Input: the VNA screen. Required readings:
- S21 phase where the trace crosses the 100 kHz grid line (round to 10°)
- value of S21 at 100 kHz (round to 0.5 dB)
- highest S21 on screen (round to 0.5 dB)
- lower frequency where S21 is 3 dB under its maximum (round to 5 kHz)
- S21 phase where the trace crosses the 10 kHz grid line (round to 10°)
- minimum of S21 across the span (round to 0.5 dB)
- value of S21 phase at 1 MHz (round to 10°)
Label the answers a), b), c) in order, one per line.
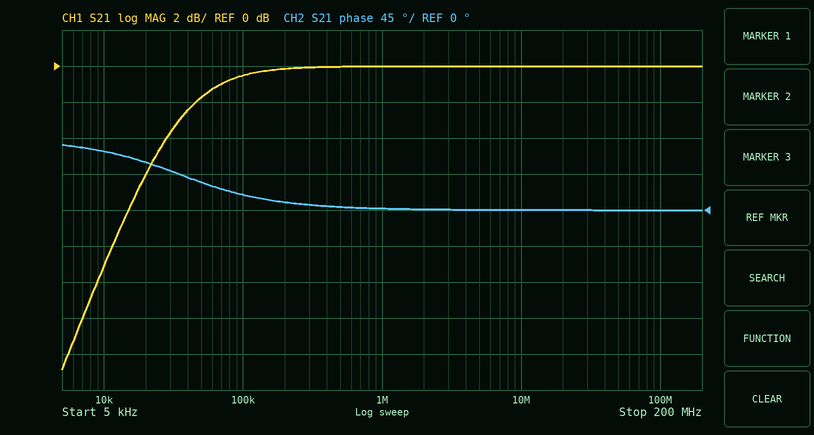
a) 20°
b) -0.5 dB
c) 0.0 dB
d) 35 kHz
e) 70°
f) -17.0 dB
g) 0°
